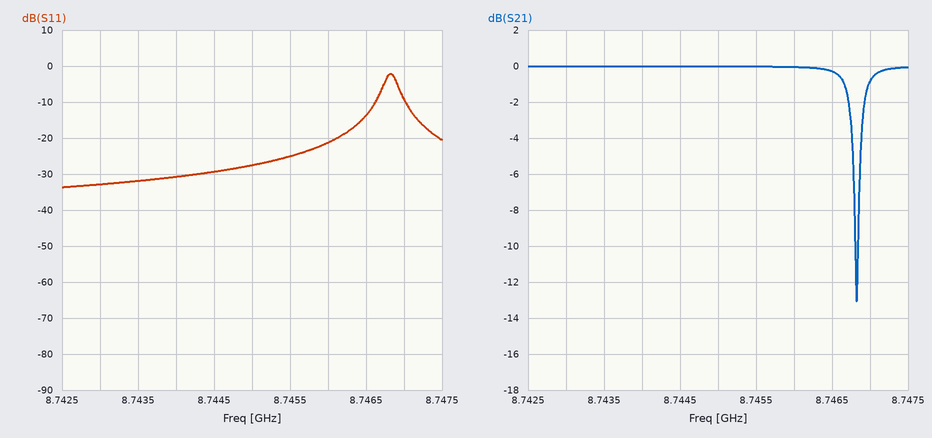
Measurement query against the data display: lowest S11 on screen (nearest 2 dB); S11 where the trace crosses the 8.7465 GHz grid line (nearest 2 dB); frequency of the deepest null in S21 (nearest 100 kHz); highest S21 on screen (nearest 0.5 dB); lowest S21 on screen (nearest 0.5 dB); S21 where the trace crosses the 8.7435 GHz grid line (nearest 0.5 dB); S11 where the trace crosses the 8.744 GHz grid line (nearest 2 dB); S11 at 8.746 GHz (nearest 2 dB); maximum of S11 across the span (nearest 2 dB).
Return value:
-34 dB
-14 dB
8.7468 GHz
0.0 dB
-13.0 dB
0.0 dB
-30 dB
-22 dB
-2 dB
